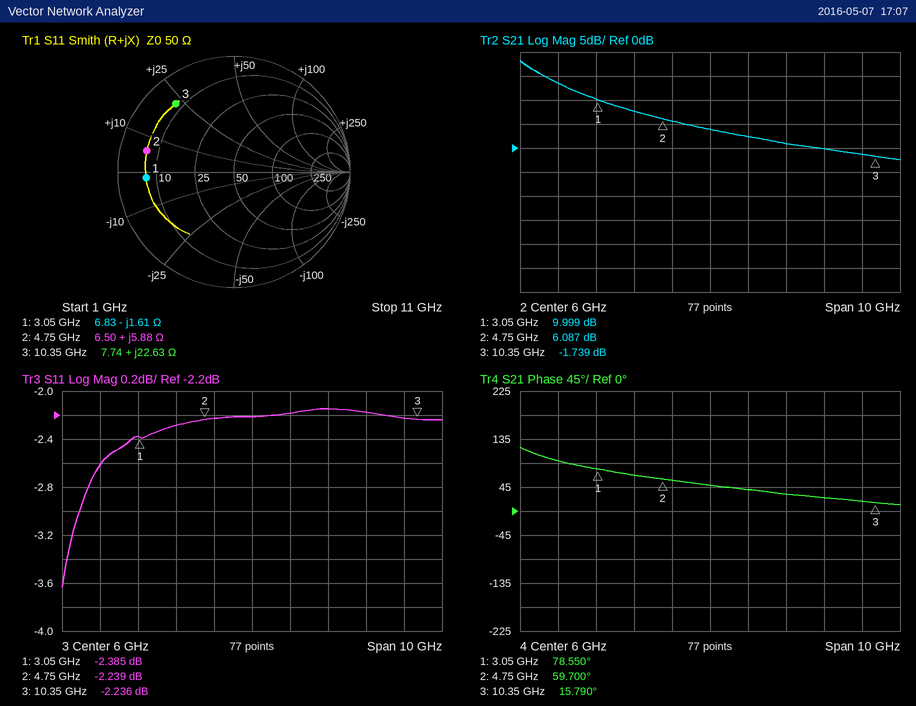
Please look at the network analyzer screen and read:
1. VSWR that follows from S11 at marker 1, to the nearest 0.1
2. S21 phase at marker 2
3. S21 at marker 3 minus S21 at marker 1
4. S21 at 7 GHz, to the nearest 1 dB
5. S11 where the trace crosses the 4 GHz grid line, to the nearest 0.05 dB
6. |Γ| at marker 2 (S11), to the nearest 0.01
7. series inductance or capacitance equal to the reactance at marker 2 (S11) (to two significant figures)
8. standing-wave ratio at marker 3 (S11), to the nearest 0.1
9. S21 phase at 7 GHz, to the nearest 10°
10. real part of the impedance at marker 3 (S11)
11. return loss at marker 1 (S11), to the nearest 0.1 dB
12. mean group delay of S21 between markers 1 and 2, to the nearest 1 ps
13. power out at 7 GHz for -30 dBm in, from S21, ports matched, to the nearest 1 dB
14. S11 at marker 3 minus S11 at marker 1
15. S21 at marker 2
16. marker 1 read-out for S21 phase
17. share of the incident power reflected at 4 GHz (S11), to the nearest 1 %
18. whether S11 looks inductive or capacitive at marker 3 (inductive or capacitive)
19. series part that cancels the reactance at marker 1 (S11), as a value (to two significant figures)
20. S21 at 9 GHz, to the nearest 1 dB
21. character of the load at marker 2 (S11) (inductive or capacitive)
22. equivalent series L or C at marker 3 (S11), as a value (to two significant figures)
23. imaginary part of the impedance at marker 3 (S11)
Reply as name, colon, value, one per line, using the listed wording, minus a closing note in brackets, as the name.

VSWR that follows from S11 at marker 1, to the nearest 0.1: 7.3
S21 phase at marker 2: 59.700°
S21 at marker 3 minus S21 at marker 1: -11.738 dB
S21 at 7 GHz, to the nearest 1 dB: 2 dB
S11 where the trace crosses the 4 GHz grid line, to the nearest 0.05 dB: -2.30 dB
|Γ| at marker 2 (S11), to the nearest 0.01: 0.77
series inductance or capacitance equal to the reactance at marker 2 (S11): 200 pH
standing-wave ratio at marker 3 (S11), to the nearest 0.1: 7.8
S21 phase at 7 GHz, to the nearest 10°: 40°
real part of the impedance at marker 3: 7.74 Ω
return loss at marker 1 (S11), to the nearest 0.1 dB: 2.4 dB
mean group delay of S21 between markers 1 and 2, to the nearest 1 ps: 31 ps
power out at 7 GHz for -30 dBm in, from S21, ports matched, to the nearest 1 dB: -28 dBm
S11 at marker 3 minus S11 at marker 1: 0.149 dB
S21 at marker 2: 6.087 dB
marker 1 read-out for S21 phase: 78.550°
share of the incident power reflected at 4 GHz (S11), to the nearest 1 %: 59 %
whether S11 looks inductive or capacitive at marker 3: inductive
series part that cancels the reactance at marker 1 (S11), as a value: 84 pH
S21 at 9 GHz, to the nearest 1 dB: 0 dB
character of the load at marker 2 (S11): inductive
equivalent series L or C at marker 3 (S11), as a value: 350 pH
imaginary part of the impedance at marker 3: +22.63 Ω
